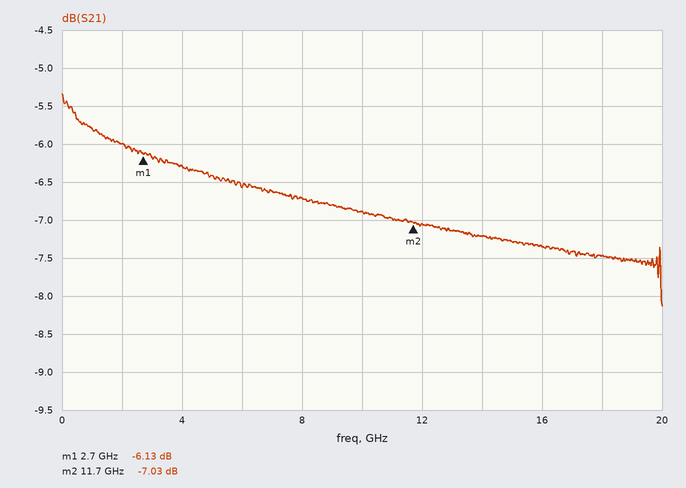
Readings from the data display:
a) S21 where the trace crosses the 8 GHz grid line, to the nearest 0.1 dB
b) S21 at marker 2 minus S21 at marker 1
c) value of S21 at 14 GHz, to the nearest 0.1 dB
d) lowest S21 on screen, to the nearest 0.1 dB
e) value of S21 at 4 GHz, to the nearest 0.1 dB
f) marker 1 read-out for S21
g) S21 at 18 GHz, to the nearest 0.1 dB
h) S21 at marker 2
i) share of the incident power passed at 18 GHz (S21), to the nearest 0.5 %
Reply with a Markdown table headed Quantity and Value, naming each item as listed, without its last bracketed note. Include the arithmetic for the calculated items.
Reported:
| Quantity | Value |
|---|---|
| S21 where the trace crosses the 8 GHz grid line, to the nearest 0.1 dB | -6.7 dB |
| S21 at marker 2 minus S21 at marker 1 | -7.03 − (-6.13) = -0.90 dB |
| value of S21 at 14 GHz, to the nearest 0.1 dB | -7.2 dB |
| lowest S21 on screen, to the nearest 0.1 dB | -8.1 dB |
| value of S21 at 4 GHz, to the nearest 0.1 dB | -6.3 dB |
| marker 1 read-out for S21 | -6.13 dB |
| S21 at 18 GHz, to the nearest 0.1 dB | -7.5 dB |
| S21 at marker 2 | -7.03 dB |
| share of the incident power passed at 18 GHz (S21), to the nearest 0.5 % | 10^(-7.5/10) ≈ 17.8 %, so 18.0 % to the nearest 0.5 % |
